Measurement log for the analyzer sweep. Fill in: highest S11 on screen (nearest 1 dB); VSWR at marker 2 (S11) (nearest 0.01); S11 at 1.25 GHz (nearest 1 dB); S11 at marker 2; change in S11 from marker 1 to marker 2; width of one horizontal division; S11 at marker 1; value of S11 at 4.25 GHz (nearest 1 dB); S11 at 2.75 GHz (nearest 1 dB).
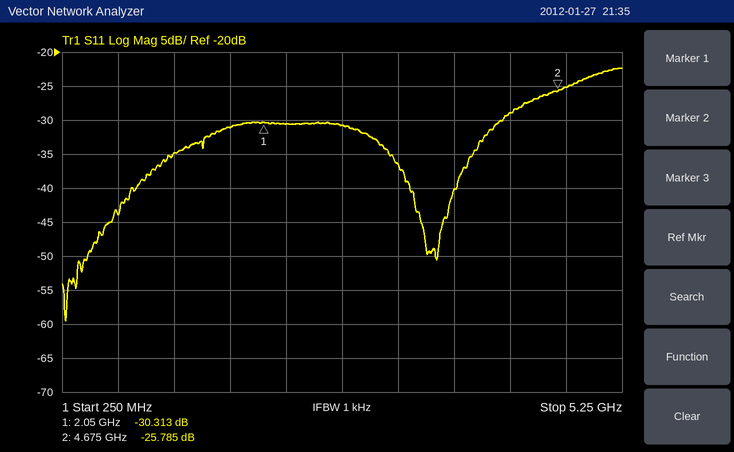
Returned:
-22 dB
1.11
-35 dB
-25.785 dB
4.528 dB
500 MHz
-30.313 dB
-29 dB
-31 dB
